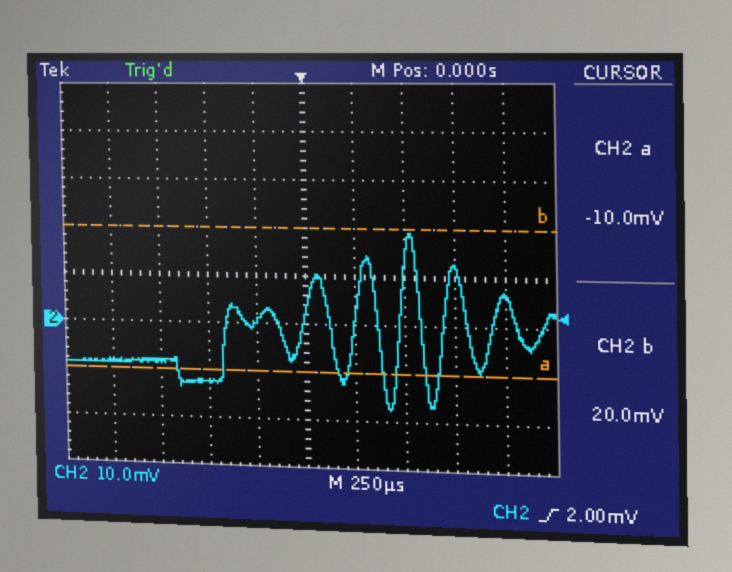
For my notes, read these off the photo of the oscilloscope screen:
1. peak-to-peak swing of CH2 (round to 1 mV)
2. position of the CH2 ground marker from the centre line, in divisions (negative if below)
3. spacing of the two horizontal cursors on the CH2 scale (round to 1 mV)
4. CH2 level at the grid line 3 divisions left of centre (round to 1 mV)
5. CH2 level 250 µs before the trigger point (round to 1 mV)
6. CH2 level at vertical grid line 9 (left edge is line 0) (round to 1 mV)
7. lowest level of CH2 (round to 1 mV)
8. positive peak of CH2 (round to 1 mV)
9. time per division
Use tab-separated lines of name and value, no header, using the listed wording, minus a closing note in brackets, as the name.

peak-to-peak swing of CH2	37 mV
position of the CH2 ground marker from the centre line, in divisions	-1.0 div
spacing of the two horizontal cursors on the CH2 scale	30 mV
CH2 level at the grid line 3 divisions left of centre	-8 mV
CH2 level 250 µs before the trigger point	0 mV
CH2 level at vertical grid line 9 (left edge is line 0)	6 mV
lowest level of CH2	-18 mV
positive peak of CH2	19 mV
time per division	250 µs
